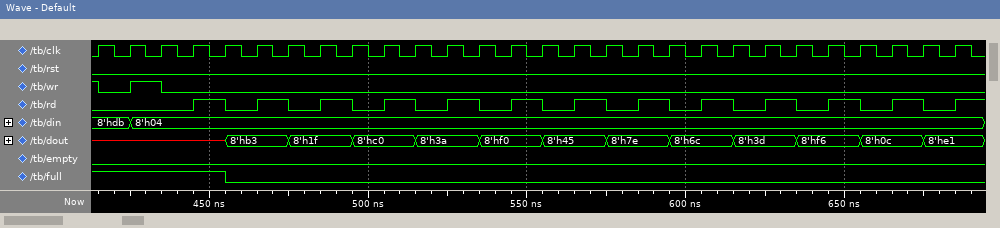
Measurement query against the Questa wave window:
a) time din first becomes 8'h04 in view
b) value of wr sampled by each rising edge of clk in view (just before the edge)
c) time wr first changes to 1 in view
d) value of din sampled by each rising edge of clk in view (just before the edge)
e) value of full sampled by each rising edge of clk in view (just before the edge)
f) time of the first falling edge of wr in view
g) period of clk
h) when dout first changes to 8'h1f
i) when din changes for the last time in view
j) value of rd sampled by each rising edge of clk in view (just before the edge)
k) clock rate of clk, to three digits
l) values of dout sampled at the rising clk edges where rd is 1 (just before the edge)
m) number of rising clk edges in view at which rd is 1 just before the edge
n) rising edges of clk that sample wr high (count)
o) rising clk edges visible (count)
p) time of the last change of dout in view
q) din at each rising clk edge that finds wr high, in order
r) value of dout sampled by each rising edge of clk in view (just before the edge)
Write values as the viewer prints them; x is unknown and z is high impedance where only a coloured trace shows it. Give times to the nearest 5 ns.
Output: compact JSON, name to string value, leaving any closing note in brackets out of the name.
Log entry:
{"time din first becomes 8'h04 in view": "425 ns", "value of wr sampled by each rising edge of clk in view": "1 0 1 0 0 0 0 0 0 0 0 0 0 0 0 0 0 0 0 0 0 0 0 0 0 0 0 0", "time wr first changes to 1 in view": "425 ns", "value of din sampled by each rising edge of clk in view": "8'hdb, 8'hdb, 8'h04, 8'h04, 8'h04, 8'h04, 8'h04, 8'h04, 8'h04, 8'h04, 8'h04, 8'h04, 8'h04, 8'h04, 8'h04, 8'h04, 8'h04, 8'h04, 8'h04, 8'h04, 8'h04, 8'h04, 8'h04, 8'h04, 8'h04, 8'h04, 8'h04, 8'h04", "value of full sampled by each rising edge of clk in view": "1 1 1 1 1 0 0 0 0 0 0 0 0 0 0 0 0 0 0 0 0 0 0 0 0 0 0 0", "time of the first falling edge of wr in view": "415 ns", "period of clk": "10 ns", "when dout first changes to 8'h1f": "475 ns", "when din changes for the last time in view": "425 ns", "value of rd sampled by each rising edge of clk in view": "0 0 0 0 1 0 1 0 1 0 1 0 1 0 1 0 1 0 1 0 1 0 1 0 1 0 1 0", "clock rate of clk, to three digits": "100 MHz", "values of dout sampled at the rising clk edges where rd is 1": "x, 8'hb3, 8'h1f, 8'hc0, 8'h3a, 8'hf0, 8'h45, 8'h7e, 8'h6c, 8'h3d, 8'hf6, 8'h0c", "number of rising clk edges in view at which rd is 1 just before the edge": "12", "rising edges of clk that sample wr high": "2", "rising clk edges visible": "28", "time of the last change of dout in view": "675 ns", "din at each rising clk edge that finds wr high, in order": "8'hdb, 8'h04", "value of dout sampled by each rising edge of clk in view": "x, x, x, x, x, 8'hb3, 8'hb3, 8'h1f, 8'h1f, 8'hc0, 8'hc0, 8'h3a, 8'h3a, 8'hf0, 8'hf0, 8'h45, 8'h45, 8'h7e, 8'h7e, 8'h6c, 8'h6c, 8'h3d, 8'h3d, 8'hf6, 8'hf6, 8'h0c, 8'h0c, 8'he1"}
